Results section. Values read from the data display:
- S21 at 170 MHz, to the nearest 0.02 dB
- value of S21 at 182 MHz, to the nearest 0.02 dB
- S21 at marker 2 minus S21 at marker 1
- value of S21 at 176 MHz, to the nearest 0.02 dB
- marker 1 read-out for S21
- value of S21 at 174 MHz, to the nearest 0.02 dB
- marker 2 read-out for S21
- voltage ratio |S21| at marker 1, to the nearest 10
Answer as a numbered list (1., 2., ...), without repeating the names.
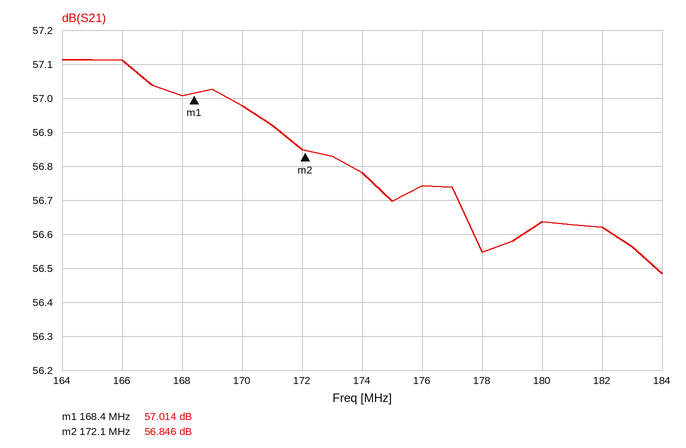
1. 56.98 dB
2. 56.62 dB
3. -0.168 dB
4. 56.74 dB
5. 57.014 dB
6. 56.78 dB
7. 56.846 dB
8. 710
